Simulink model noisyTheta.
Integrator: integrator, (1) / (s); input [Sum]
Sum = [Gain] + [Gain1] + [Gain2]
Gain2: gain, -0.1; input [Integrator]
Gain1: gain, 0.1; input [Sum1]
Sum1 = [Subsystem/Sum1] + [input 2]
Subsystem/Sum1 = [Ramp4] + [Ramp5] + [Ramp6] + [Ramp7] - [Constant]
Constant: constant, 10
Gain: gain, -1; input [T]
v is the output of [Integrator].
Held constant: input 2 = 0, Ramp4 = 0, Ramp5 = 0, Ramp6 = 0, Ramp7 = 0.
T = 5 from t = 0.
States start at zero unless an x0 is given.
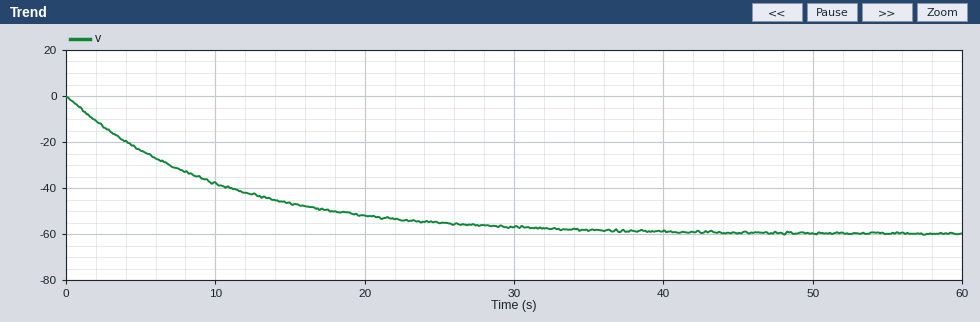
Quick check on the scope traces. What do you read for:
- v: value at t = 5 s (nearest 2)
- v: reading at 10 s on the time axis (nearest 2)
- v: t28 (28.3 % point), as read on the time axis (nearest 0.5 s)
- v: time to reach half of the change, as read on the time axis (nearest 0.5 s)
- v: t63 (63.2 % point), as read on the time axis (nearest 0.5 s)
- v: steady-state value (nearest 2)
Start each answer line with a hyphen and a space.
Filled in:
- -24
- -38
- 3.5 s
- 7.0 s
- 10.0 s
- -60
